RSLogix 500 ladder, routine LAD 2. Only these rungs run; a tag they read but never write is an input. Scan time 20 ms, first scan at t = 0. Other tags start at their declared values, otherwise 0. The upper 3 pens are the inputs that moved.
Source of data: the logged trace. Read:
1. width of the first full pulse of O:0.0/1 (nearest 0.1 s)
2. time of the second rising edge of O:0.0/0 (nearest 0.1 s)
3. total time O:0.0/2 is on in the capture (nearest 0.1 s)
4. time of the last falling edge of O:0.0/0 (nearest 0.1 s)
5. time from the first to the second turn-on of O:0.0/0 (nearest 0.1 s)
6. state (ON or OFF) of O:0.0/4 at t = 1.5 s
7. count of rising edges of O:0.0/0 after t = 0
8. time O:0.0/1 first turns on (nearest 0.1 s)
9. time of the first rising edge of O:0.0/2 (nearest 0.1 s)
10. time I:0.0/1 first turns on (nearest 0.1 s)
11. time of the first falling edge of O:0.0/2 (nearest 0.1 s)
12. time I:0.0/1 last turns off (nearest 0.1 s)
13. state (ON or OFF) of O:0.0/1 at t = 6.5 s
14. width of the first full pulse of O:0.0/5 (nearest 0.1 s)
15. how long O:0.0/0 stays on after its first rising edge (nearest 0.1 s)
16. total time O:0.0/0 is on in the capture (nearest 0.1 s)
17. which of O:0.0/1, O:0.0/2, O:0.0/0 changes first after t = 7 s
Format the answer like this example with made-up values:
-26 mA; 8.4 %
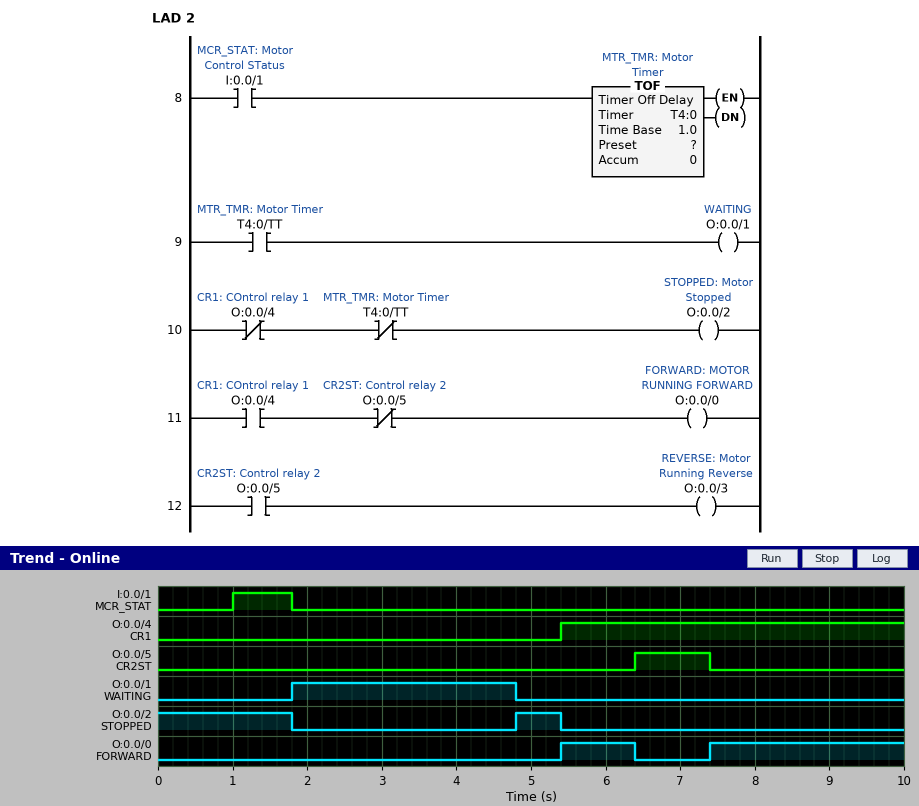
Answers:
3.0 s; 7.4 s; 2.4 s; 6.4 s; 2.0 s; OFF; 2; 1.8 s; 4.8 s; 1.0 s; 1.8 s; 1.8 s; OFF; 1.0 s; 1.0 s; 3.6 s; O:0.0/0
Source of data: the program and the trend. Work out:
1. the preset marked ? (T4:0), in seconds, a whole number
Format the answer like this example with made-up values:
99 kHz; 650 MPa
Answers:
3 s
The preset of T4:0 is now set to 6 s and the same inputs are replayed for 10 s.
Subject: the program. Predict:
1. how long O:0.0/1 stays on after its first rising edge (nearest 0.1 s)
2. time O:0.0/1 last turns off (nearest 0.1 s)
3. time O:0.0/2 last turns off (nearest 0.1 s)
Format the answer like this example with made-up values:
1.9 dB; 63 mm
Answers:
6.0 s; 7.8 s; 1.8 s
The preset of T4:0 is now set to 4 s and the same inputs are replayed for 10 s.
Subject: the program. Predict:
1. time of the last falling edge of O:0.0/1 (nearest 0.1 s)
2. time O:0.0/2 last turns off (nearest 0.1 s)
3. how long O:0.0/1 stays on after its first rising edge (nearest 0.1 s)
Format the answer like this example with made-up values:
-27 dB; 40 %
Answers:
5.8 s; 1.8 s; 4.0 s
